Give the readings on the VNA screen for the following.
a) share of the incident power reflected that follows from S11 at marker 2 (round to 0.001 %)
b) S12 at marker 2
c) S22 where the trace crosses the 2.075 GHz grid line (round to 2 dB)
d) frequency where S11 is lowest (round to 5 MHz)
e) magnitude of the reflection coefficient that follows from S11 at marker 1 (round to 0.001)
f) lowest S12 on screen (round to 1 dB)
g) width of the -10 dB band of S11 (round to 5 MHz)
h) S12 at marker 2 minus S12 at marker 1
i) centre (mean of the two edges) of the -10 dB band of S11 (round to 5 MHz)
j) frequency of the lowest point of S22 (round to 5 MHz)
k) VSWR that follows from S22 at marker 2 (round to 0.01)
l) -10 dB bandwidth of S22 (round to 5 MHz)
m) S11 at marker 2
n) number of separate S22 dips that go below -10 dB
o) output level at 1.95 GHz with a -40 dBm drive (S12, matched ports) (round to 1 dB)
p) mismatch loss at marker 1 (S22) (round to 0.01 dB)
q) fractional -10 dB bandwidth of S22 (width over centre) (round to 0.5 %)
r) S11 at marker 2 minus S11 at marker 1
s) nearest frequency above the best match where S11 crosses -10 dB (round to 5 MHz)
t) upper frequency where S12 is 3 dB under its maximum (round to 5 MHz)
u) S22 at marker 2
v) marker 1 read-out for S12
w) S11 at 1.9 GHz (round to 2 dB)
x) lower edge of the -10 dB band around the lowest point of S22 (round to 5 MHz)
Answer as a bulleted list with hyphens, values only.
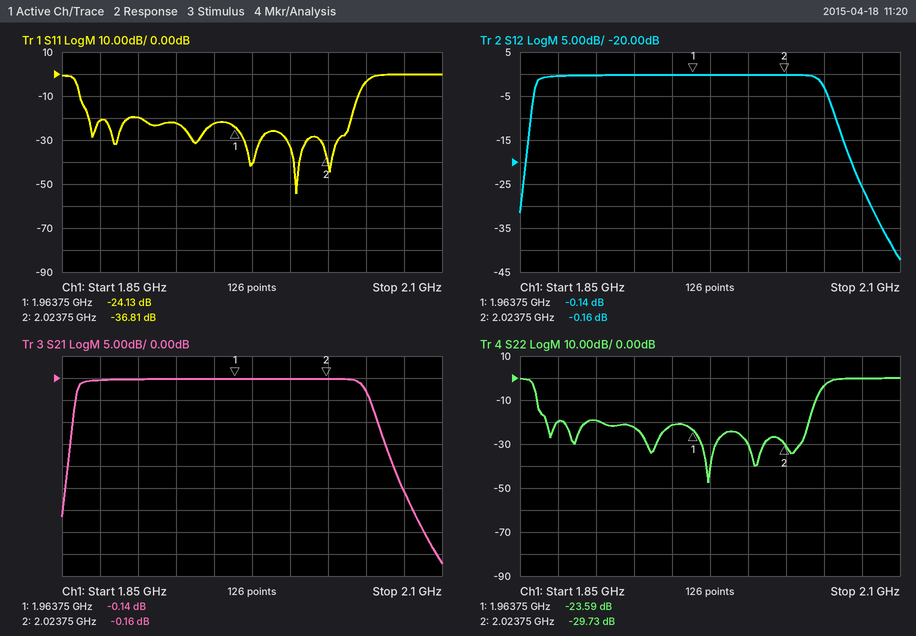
- 0.021 %
- -0.16 dB
- 0 dB
- 2.005 GHz
- 0.062
- -42 dB
- 185 MHz
- -0.02 dB
- 1.955 GHz
- 1.975 GHz
- 1.07
- 185 MHz
- -36.81 dB
- 6
- -40 dBm
- 0.02 dB
- 9.5 %
- -12.68 dB
- 2.045 GHz
- 2.050 GHz
- -29.73 dB
- -0.14 dB
- -20 dB
- 1.860 GHz
